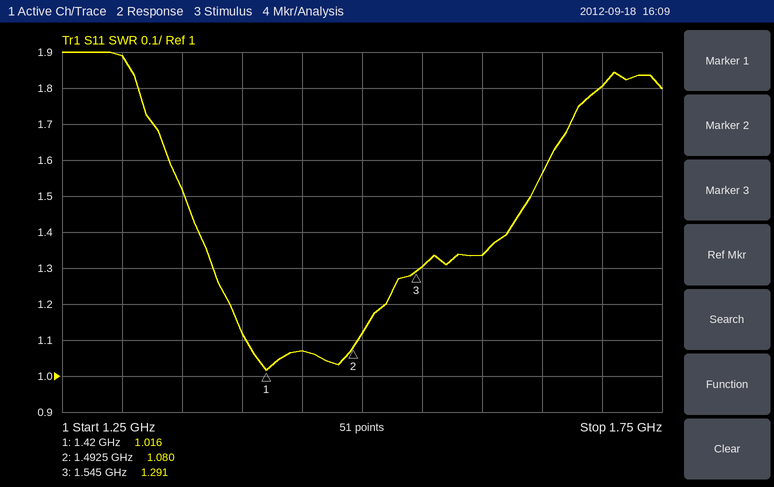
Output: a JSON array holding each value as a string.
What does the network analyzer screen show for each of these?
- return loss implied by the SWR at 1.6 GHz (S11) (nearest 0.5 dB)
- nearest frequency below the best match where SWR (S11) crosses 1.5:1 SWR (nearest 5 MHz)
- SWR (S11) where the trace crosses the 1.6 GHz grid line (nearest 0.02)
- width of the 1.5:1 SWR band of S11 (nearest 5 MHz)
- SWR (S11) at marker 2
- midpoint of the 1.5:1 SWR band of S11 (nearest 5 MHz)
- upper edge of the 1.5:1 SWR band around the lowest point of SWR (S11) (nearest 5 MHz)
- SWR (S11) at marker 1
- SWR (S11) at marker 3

["17.0 dB", "1.350 GHz", "1.34", "290 MHz", "1.080", "1.495 GHz", "1.640 GHz", "1.016", "1.291"]
